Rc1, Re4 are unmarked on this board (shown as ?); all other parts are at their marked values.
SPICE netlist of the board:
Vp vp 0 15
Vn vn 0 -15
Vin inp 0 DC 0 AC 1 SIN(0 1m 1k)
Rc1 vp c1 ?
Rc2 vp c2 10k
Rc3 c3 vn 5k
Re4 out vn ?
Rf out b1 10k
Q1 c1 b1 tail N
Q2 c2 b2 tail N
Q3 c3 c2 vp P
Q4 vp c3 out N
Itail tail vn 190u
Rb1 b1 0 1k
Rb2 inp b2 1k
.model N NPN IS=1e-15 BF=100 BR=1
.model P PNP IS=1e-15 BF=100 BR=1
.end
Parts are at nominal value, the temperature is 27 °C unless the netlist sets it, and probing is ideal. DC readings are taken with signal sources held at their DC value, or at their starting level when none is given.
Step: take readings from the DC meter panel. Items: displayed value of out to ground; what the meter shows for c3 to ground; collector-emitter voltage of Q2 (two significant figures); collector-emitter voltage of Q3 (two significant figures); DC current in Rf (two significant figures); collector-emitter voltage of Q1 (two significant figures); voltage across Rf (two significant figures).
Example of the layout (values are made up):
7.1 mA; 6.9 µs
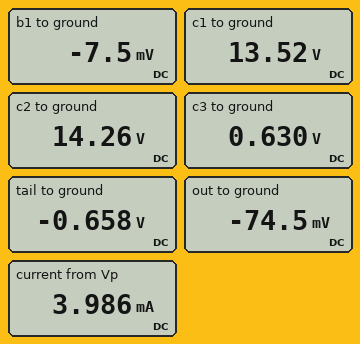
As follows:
-74.5 mV; 0.630 V; 15 V; -14 V; 6.7 µA; 14 V; 67 mV
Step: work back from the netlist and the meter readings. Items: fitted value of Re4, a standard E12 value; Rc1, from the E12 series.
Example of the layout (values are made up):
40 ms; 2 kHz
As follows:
22 kΩ; 18 kΩ
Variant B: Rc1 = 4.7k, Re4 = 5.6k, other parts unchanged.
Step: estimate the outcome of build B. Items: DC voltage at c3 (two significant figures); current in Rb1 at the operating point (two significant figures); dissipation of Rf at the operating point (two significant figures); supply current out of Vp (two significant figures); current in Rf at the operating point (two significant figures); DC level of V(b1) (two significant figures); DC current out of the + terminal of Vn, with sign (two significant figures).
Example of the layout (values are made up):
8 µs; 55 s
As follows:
660 mV; 7.7 µA; 470 nW; 6.0 mA; 6.9 µA; -7.7 mV; -6.0 mA
